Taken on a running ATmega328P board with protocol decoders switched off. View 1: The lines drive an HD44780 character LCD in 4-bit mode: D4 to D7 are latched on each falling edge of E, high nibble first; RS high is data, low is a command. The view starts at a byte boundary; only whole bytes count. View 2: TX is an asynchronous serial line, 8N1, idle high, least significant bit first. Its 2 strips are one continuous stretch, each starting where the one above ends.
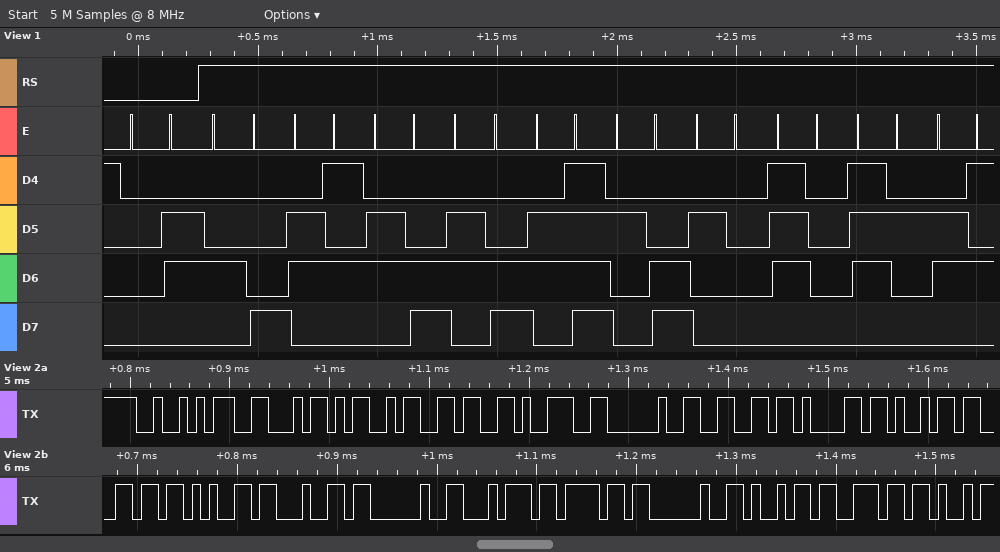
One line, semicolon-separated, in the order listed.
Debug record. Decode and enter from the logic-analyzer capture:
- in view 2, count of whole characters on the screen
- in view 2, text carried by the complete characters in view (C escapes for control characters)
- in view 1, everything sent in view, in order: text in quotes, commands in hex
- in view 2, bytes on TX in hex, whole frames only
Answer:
18; "RFM69 failed to in"; 0x06 "Hello, pre"; 0x52 0x46 0x4D 0x36 0x39 0x20 0x66 0x61 0x69 0x6C 0x65 0x64 0x20 0x74 0x6F 0x20 0x69 0x6E
